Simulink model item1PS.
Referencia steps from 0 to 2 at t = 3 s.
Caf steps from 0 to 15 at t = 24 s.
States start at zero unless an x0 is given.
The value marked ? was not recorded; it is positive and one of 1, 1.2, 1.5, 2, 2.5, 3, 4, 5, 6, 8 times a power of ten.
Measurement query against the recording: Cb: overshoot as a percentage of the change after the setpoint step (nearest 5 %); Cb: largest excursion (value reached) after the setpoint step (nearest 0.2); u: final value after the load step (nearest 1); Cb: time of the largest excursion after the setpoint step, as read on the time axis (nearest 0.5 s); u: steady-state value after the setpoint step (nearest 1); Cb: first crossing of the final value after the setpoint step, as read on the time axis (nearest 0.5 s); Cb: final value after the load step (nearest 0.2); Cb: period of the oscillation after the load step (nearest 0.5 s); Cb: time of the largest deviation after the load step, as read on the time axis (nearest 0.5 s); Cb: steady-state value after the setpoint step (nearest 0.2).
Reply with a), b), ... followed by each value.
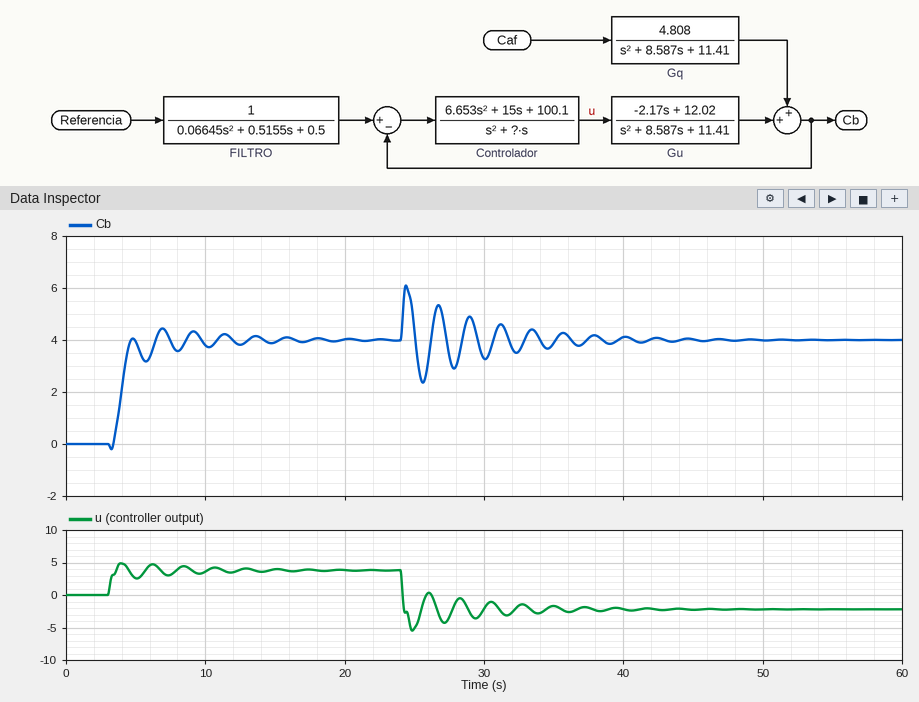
a) 10 %
b) 4.4
c) -2
d) 7.0 s
e) 4
f) 4.5 s
g) 4.0
h) 2.5 s
i) 24.5 s
j) 4.0
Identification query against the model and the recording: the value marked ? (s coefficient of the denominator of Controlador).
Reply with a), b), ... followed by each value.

a) 12
